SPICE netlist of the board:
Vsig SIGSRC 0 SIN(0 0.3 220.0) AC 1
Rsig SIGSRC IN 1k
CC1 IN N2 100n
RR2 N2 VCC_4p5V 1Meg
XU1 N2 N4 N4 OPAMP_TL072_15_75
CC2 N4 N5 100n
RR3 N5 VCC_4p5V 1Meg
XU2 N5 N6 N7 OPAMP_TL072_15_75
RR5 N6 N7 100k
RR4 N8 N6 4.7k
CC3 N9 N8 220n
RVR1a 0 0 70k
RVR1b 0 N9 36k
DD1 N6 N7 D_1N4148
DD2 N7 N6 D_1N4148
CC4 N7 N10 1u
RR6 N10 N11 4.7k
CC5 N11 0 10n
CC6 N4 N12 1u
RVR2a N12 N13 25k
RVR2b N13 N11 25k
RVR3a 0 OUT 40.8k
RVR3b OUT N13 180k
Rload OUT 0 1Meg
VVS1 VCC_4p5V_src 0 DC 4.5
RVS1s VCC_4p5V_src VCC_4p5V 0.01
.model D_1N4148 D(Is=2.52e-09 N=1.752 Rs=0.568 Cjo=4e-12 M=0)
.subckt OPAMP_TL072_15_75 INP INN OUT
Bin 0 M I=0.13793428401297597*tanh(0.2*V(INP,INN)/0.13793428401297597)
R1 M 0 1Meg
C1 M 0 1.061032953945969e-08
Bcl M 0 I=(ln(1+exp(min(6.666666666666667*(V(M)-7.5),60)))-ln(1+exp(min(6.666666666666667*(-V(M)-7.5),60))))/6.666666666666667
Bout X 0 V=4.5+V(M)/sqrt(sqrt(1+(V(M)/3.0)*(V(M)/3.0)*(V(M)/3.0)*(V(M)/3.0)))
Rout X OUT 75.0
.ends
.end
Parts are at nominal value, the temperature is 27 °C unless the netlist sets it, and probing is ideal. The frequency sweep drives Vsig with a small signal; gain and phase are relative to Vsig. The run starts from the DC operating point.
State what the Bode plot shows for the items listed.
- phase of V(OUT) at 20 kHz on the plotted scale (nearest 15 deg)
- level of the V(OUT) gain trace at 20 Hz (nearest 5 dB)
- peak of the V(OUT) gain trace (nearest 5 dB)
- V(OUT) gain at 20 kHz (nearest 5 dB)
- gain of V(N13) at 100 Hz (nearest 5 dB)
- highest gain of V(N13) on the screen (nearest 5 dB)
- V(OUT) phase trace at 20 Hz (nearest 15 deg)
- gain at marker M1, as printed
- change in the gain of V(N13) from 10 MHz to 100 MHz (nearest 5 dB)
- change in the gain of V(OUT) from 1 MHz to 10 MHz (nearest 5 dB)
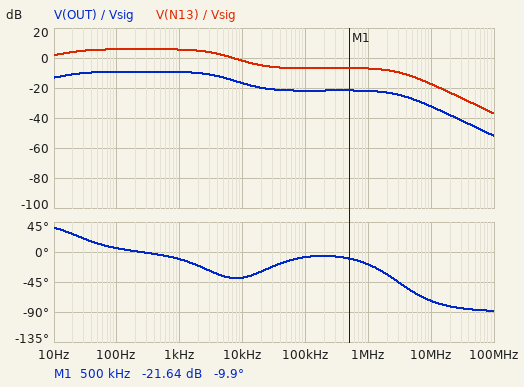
-30 deg
-10 dB
-10 dB
-20 dB
5 dB
5 dB
30 deg
-21.64 dB
-20 dB
-10 dB
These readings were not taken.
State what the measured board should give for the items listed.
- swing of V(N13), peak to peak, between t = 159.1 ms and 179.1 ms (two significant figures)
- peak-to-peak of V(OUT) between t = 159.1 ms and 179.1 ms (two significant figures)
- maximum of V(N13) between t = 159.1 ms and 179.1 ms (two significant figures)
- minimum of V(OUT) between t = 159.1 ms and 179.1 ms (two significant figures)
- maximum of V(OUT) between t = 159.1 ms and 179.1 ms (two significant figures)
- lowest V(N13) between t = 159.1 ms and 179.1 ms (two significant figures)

850 mV
150 mV
420 mV
-76 mV
76 mV
-420 mV
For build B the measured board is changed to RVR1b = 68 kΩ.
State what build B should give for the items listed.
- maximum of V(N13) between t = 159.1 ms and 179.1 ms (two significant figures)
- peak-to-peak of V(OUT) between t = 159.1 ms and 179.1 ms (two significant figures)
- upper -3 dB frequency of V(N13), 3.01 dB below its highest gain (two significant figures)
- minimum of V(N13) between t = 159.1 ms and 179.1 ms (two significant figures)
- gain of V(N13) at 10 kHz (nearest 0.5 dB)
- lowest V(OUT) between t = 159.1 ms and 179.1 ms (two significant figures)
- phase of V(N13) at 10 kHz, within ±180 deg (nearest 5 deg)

400 mV
140 mV
4.2 kHz
-400 mV
-3.5 dB
-72 mV
-30 deg
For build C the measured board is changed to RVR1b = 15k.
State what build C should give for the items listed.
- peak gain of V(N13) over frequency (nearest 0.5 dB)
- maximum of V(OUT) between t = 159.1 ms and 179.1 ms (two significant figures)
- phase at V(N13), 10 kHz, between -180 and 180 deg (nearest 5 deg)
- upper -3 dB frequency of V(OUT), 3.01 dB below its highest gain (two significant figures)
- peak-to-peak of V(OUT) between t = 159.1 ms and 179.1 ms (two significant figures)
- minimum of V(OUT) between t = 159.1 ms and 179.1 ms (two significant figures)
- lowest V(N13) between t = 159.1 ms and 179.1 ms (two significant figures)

9.5 dB
79 mV
-50 deg
3.9 kHz
160 mV
-79 mV
-440 mV
